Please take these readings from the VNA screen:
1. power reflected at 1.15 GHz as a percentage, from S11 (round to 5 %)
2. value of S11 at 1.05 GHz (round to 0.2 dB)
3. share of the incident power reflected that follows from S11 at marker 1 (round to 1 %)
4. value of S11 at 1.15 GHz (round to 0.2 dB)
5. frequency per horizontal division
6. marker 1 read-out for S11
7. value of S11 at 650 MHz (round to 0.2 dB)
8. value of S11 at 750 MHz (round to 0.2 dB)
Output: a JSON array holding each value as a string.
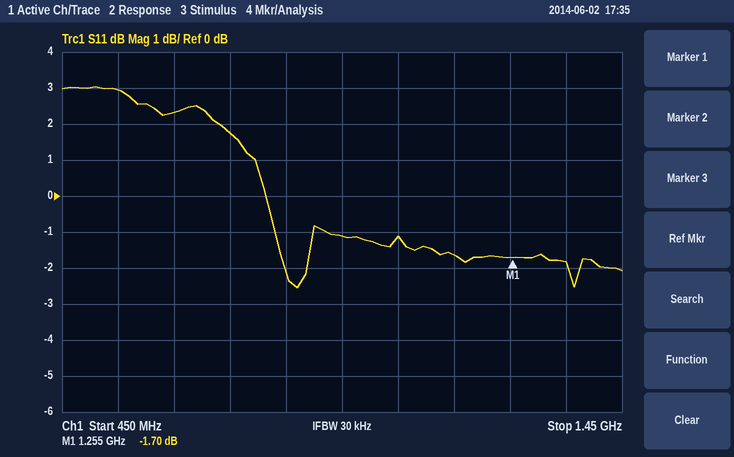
["70 %", "-1.2 dB", "68 %", "-1.6 dB", "100 MHz", "-1.70 dB", "2.4 dB", "1.8 dB"]
